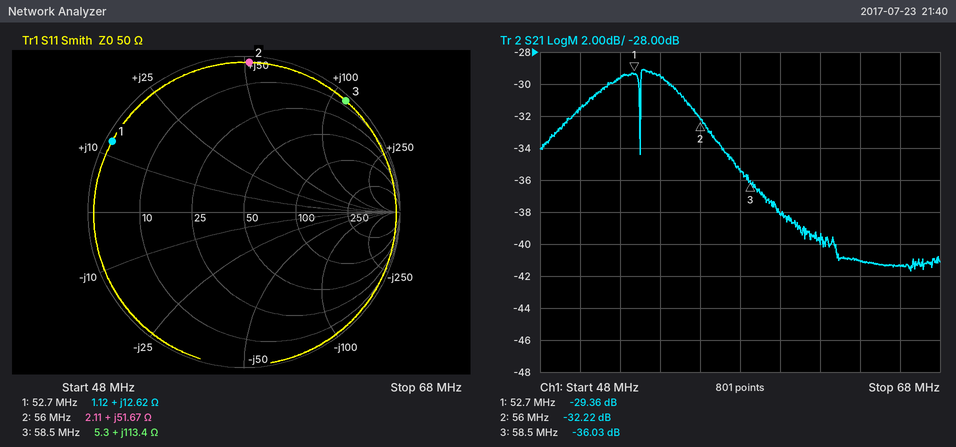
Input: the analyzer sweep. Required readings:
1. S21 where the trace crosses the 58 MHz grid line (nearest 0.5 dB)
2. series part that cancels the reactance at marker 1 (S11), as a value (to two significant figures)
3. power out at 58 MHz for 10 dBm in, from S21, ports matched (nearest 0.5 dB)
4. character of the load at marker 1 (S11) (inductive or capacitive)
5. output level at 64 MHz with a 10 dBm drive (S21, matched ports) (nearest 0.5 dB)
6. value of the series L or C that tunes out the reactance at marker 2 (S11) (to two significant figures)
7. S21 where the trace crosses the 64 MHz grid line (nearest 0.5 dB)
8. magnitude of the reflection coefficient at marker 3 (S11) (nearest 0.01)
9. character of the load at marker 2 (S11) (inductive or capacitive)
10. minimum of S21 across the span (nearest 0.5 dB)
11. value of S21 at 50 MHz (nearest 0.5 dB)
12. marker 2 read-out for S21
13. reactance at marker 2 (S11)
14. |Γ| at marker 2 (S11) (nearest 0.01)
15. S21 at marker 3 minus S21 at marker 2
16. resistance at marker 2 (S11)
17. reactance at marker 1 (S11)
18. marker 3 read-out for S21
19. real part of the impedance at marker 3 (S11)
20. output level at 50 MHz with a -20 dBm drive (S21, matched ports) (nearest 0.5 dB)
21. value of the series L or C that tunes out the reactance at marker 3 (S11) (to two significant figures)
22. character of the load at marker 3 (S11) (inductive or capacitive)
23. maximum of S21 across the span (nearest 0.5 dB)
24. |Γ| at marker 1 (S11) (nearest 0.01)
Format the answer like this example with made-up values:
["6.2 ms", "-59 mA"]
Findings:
["-35.5 dB", "240 pF", "-25.5 dBm", "inductive", "-31.0 dBm", "55 pF", "-41.0 dB", "0.97", "inductive", "-41.5 dB", "-31.5 dB", "-32.22 dB", "+51.67 Ω", "0.96", "-3.81 dB", "2.11 Ω", "+12.62 Ω", "-36.03 dB", "5.3 Ω", "-51.5 dBm", "24 pF", "inductive", "-29.0 dB", "0.96"]
